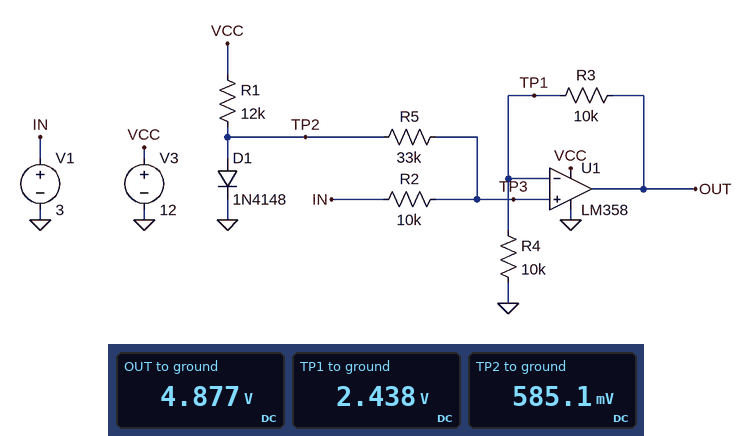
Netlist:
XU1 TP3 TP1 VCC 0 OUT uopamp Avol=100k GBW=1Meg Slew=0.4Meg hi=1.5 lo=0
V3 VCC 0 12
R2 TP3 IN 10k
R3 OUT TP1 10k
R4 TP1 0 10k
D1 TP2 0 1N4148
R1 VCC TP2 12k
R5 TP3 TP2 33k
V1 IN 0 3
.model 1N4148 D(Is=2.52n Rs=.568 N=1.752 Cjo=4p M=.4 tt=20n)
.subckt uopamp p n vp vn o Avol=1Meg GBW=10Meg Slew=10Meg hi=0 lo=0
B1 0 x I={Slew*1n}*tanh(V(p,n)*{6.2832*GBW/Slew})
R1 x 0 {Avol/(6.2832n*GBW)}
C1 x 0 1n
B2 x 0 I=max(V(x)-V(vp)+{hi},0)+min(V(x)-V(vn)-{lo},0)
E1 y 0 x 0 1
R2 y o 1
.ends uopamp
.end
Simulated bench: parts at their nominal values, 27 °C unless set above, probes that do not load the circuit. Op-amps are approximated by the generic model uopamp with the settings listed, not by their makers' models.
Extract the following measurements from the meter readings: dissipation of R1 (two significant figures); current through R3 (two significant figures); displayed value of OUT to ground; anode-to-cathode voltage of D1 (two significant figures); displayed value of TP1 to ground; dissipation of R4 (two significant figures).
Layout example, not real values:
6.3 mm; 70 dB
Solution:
11 mW; 240 µA; 4.877 V; 590 mV; 2.438 V; 590 µW
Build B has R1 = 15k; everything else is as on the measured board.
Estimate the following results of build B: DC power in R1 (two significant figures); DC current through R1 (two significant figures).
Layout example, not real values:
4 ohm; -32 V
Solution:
8.7 mW; 760 µA
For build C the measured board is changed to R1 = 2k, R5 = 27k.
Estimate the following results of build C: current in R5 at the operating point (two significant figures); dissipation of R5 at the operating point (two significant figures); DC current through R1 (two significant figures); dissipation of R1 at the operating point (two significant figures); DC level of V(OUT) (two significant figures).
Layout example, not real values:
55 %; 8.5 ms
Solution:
63 µA; 110 µW; 5.7 mA; 64 mW; 4.7 V
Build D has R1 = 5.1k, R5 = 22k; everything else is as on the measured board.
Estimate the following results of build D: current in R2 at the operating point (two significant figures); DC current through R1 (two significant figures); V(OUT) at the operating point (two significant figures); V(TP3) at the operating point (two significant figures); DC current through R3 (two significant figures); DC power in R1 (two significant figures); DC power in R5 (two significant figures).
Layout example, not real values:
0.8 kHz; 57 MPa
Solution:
74 µA; 2.2 mA; 4.5 V; 2.3 V; 230 µA; 25 mW; 120 µW
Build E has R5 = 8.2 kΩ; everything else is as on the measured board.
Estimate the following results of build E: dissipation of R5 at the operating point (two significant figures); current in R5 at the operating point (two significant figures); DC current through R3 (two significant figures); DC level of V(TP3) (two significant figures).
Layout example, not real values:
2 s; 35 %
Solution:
140 µW; 130 µA; 170 µA; 1.7 V
